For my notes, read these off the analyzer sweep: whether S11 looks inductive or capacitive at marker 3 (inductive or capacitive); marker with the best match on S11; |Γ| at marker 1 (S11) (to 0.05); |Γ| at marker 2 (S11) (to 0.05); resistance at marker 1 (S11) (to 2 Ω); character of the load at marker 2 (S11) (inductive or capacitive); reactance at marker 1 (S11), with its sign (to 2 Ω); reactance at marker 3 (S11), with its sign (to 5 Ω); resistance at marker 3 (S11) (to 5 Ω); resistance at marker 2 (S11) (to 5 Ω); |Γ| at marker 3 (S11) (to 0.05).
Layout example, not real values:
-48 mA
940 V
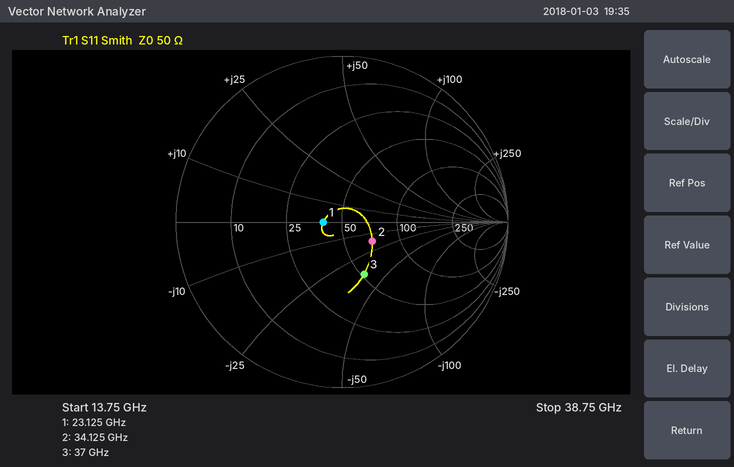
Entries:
capacitive
marker 1
0.10
0.20
40 Ω
capacitive
0 Ω
-35 Ω
50 Ω
70 Ω
0.35
